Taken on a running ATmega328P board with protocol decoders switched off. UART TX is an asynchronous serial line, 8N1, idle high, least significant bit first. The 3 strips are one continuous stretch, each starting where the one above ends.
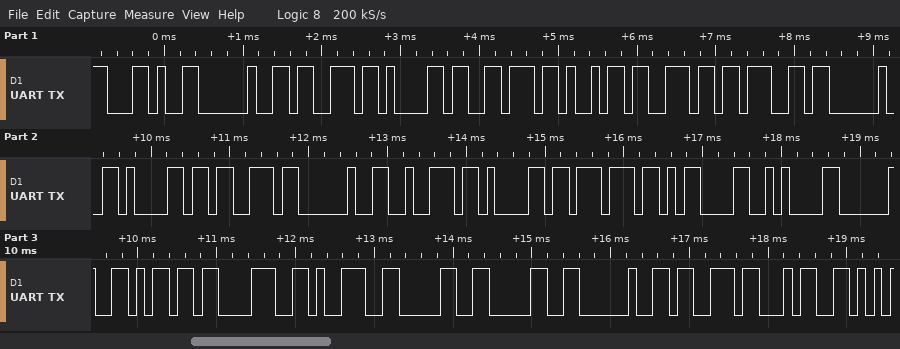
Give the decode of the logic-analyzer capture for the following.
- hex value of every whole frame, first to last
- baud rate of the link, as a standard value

2C 20 73 61 76 69 6E 67 20 61 73 20 72 61 77 0D 0A 20 6D 38 39 30 30 20 73 34
9600 baud
